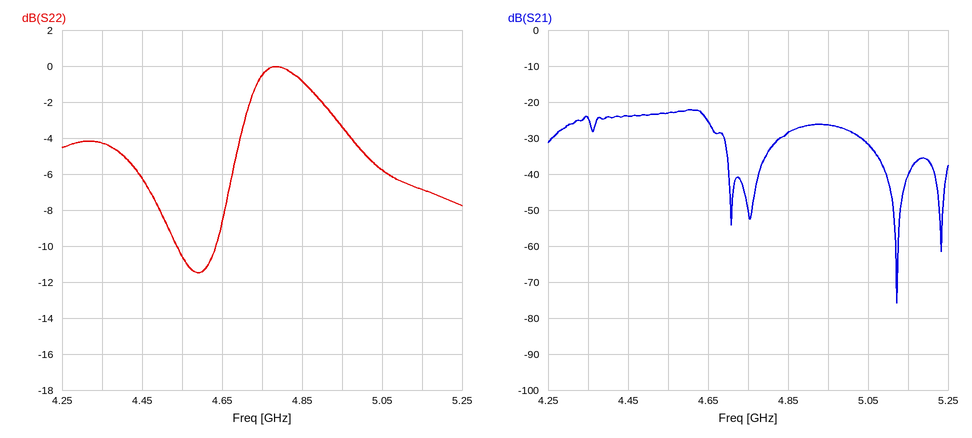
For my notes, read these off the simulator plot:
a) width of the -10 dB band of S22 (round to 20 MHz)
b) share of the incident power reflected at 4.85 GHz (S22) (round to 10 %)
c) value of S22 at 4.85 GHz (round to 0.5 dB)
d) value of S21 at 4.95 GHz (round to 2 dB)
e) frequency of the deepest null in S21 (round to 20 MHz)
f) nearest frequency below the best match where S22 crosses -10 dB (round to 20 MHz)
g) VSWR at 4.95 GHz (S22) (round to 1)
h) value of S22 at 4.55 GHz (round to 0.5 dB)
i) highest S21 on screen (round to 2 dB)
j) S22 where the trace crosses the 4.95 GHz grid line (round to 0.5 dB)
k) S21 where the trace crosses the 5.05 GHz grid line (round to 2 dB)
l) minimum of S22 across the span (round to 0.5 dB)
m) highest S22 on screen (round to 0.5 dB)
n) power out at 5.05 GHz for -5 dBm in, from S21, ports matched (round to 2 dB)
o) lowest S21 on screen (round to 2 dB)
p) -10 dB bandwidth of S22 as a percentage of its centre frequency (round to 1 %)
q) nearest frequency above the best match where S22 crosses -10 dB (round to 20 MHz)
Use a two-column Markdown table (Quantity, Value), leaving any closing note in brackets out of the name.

| Quantity | Value |
|---|---|
| width of the -10 dB band of S22 | 100 MHz |
| share of the incident power reflected at 4.85 GHz (S22) | 80 % |
| value of S22 at 4.85 GHz | -1.0 dB |
| value of S21 at 4.95 GHz | -26 dB |
| frequency of the deepest null in S21 | 5.12 GHz |
| nearest frequency below the best match where S22 crosses -10 dB | 4.54 GHz |
| VSWR at 4.95 GHz (S22) | 5 |
| value of S22 at 4.55 GHz | -10.5 dB |
| highest S21 on screen | -22 dB |
| S22 where the trace crosses the 4.95 GHz grid line | -3.5 dB |
| S21 where the trace crosses the 5.05 GHz grid line | -32 dB |
| minimum of S22 across the span | -11.5 dB |
| highest S22 on screen | 0.0 dB |
| power out at 5.05 GHz for -5 dBm in, from S21, ports matched | -36 dBm |
| lowest S21 on screen | -76 dB |
| -10 dB bandwidth of S22 as a percentage of its centre frequency | 2 % |
| nearest frequency above the best match where S22 crosses -10 dB | 4.64 GHz |
